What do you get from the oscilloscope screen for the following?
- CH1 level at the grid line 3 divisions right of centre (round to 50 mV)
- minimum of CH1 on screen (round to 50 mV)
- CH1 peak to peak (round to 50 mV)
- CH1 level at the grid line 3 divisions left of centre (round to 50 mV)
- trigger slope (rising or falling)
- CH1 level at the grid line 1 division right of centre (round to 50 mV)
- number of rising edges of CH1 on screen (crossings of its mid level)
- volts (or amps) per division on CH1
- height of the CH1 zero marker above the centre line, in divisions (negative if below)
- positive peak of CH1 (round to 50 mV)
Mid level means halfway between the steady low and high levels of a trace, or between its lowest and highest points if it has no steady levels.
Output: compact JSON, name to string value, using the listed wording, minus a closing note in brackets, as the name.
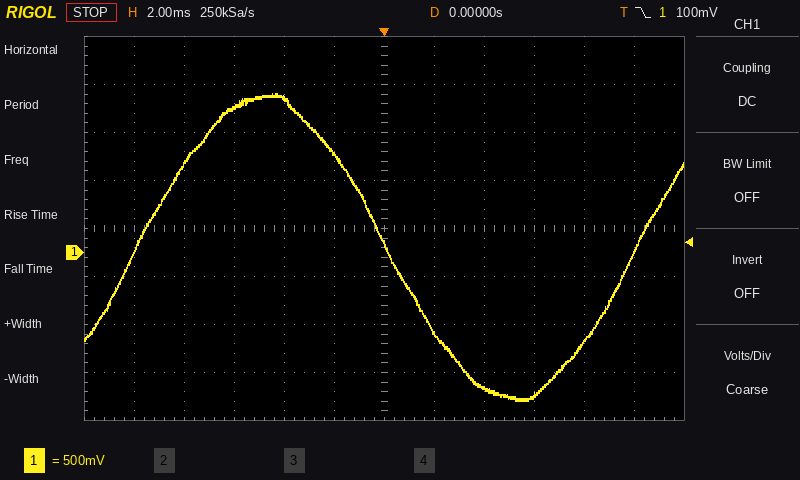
{"CH1 level at the grid line 3 divisions right of centre": "-1.50 V", "minimum of CH1 on screen": "-1.55 V", "CH1 peak to peak": "3.20 V", "CH1 level at the grid line 3 divisions left of centre": "1.50 V", "trigger slope": "falling", "CH1 level at the grid line 1 division right of centre": "-850 mV", "number of rising edges of CH1 on screen": "2", "volts (or amps) per division on CH1": "500 mV", "height of the CH1 zero marker above the centre line, in divisions": "-0.5 div", "positive peak of CH1": "1.65 V"}
